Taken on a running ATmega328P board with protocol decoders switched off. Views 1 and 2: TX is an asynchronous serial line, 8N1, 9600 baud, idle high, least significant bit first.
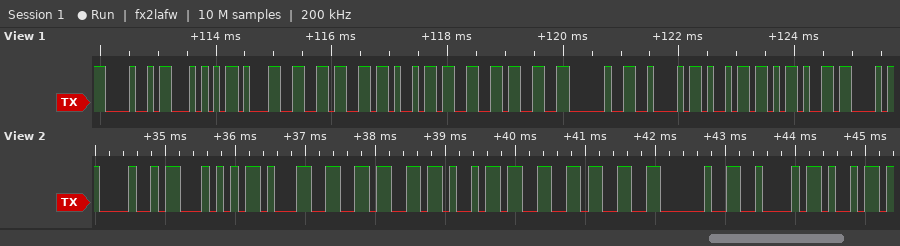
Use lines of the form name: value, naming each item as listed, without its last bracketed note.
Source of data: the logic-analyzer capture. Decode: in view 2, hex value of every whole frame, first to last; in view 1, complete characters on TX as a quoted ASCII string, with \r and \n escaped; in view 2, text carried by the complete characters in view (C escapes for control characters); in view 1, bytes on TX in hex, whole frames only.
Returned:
in view 2, hex value of every whole frame, first to last: 48 54 31 36 4B 33 33 20 42 69
in view 1, complete characters on TX as a quoted ASCII string, with \r and \n escaped: "HT16K33 Bi-C"
in view 2, text carried by the complete characters in view: "HT16K33 Bi"
in view 1, bytes on TX in hex, whole frames only: 48 54 31 36 4B 33 33 20 42 69 2D 43
